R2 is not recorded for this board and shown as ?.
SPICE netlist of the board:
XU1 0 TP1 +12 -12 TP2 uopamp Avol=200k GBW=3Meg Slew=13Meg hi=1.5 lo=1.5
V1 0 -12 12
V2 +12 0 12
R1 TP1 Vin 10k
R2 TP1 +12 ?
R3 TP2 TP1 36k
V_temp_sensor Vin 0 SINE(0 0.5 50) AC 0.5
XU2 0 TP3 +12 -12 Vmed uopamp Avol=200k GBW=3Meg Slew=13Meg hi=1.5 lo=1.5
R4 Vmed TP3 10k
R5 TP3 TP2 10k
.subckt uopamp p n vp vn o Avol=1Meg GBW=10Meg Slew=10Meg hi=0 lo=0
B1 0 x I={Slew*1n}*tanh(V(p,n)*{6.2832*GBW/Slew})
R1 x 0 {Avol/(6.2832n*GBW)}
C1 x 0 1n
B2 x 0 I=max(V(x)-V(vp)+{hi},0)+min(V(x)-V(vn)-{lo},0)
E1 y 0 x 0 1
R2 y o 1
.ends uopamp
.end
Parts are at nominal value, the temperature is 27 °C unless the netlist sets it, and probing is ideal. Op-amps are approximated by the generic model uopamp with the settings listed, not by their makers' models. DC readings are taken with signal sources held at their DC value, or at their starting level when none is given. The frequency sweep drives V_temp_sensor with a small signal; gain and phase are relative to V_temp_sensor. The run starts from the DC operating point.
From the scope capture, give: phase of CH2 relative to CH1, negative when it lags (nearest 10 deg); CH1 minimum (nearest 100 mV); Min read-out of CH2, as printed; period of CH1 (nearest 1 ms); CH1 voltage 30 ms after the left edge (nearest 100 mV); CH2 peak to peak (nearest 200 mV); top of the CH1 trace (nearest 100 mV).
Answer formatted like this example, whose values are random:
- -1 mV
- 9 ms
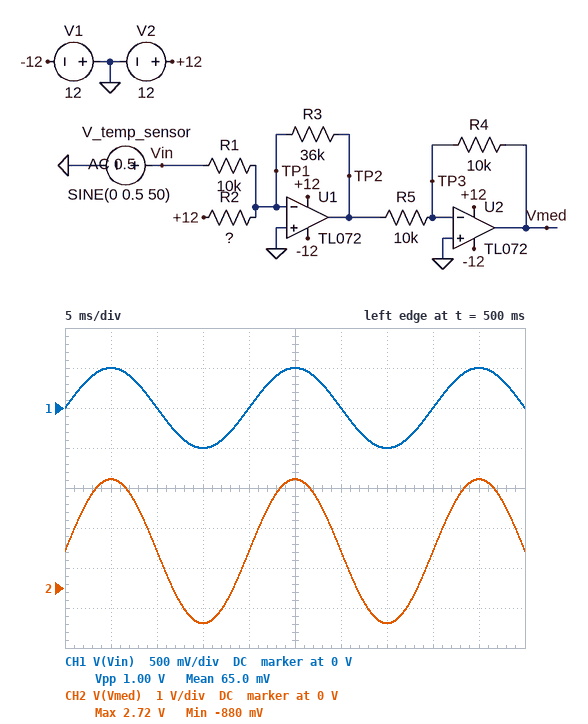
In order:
- 0 deg
- -500 mV
- -880 mV
- 20 ms
- 0 V
- 3.6 V
- 500 mV
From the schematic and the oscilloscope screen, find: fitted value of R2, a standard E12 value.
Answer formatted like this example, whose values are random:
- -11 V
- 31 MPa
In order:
- 470 kΩ
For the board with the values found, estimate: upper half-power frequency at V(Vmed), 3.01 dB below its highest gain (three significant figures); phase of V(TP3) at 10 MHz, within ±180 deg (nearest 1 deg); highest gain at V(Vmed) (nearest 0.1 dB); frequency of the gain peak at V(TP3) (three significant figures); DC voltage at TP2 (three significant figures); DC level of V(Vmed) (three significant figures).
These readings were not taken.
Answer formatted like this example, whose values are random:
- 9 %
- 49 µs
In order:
- 558 kHz
- 102 deg
- 11.1 dB
- 981 kHz
- -919 mV
- 919 mV
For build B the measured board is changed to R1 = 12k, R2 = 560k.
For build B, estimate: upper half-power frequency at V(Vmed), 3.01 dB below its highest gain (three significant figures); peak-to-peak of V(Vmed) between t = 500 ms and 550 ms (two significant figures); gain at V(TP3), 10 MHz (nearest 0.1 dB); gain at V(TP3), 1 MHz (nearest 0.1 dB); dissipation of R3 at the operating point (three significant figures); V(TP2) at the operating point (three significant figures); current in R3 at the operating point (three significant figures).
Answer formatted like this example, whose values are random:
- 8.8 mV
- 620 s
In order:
- 621 kHz
- 3.0 V
- -19.2 dB
- -6.1 dB
- 16.5 µW
- -771 mV
- 21.4 µA
